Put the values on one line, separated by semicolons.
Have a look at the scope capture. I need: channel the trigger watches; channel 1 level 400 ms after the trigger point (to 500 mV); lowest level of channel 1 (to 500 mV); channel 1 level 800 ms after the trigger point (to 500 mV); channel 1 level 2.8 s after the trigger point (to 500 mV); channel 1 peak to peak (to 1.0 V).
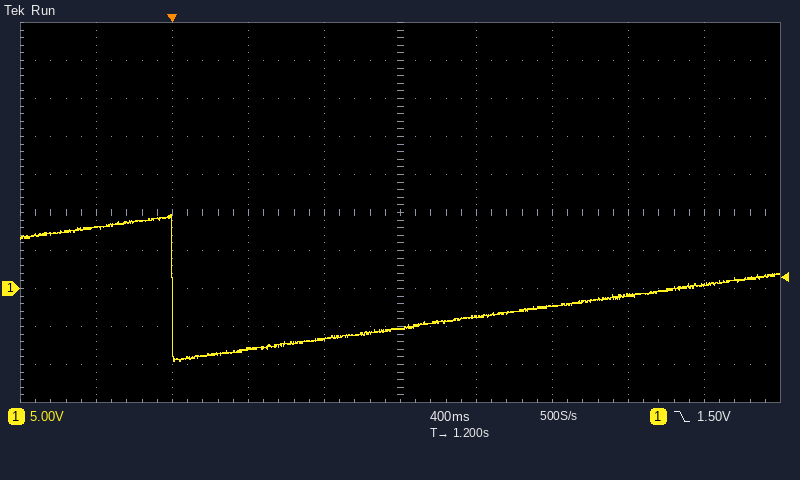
channel 1; -8.0 V; -9.5 V; -6.5 V; 500 mV; 19.0 V
